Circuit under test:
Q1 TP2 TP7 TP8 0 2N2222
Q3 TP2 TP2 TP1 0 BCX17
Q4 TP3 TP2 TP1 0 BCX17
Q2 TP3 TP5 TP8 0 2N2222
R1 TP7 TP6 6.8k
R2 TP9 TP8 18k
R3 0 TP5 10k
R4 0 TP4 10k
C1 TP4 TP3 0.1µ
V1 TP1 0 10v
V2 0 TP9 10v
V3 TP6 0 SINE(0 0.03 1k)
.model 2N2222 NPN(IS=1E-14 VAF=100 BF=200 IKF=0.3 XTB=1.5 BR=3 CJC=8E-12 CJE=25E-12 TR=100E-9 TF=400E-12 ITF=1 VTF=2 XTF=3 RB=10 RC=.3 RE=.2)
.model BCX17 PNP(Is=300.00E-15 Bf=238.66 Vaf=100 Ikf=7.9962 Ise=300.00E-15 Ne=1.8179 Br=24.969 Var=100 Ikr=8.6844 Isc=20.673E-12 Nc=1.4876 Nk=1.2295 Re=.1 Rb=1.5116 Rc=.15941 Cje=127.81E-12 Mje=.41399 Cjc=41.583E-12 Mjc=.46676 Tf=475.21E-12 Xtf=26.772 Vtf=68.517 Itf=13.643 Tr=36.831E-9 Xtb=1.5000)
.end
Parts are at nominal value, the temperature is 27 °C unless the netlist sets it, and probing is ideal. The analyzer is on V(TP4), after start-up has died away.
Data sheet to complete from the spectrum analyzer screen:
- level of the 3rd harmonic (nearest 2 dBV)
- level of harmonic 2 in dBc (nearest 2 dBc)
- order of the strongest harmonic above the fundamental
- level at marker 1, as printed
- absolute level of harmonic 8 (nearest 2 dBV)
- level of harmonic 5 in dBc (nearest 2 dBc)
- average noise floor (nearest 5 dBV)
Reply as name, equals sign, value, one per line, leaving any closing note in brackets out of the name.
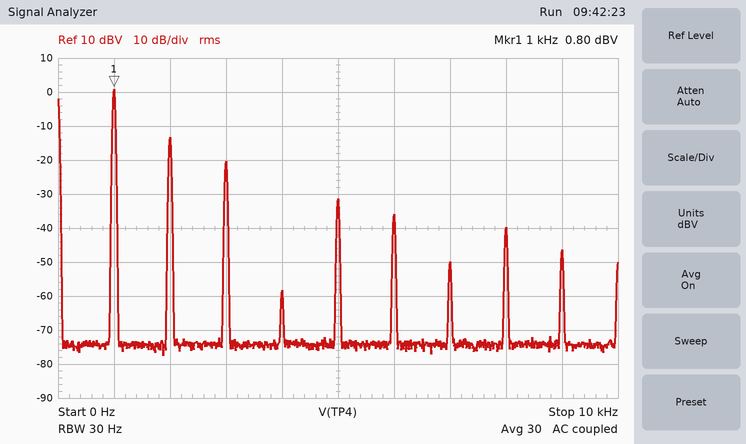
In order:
level of the 3rd harmonic = -20 dBV
level of harmonic 2 in dBc = -14 dBc
order of the strongest harmonic above the fundamental = 2
level at marker 1, as printed = 0.80 dBV
absolute level of harmonic 8 = -40 dBV
level of harmonic 5 in dBc = -32 dBc
average noise floor = -75 dBV
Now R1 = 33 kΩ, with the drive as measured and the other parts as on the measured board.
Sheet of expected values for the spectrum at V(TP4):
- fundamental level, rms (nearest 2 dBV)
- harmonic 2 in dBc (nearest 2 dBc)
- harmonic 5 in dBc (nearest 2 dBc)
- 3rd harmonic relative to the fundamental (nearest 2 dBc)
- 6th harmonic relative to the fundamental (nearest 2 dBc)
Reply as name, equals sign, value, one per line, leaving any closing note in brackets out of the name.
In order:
fundamental level, rms = -14 dBV
harmonic 2 in dBc = -4 dBc
harmonic 5 in dBc = -36 dBc
3rd harmonic relative to the fundamental = -10 dBc
6th harmonic relative to the fundamental = -26 dBc
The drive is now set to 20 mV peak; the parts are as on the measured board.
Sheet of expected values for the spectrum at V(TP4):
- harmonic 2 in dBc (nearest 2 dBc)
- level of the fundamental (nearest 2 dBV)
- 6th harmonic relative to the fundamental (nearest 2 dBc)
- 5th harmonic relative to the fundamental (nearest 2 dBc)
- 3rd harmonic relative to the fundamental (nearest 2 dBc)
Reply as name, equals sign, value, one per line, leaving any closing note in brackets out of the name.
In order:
harmonic 2 in dBc = -12 dBc
level of the fundamental = -4 dBV
6th harmonic relative to the fundamental = -54 dBc
5th harmonic relative to the fundamental = -30 dBc
3rd harmonic relative to the fundamental = -22 dBc
